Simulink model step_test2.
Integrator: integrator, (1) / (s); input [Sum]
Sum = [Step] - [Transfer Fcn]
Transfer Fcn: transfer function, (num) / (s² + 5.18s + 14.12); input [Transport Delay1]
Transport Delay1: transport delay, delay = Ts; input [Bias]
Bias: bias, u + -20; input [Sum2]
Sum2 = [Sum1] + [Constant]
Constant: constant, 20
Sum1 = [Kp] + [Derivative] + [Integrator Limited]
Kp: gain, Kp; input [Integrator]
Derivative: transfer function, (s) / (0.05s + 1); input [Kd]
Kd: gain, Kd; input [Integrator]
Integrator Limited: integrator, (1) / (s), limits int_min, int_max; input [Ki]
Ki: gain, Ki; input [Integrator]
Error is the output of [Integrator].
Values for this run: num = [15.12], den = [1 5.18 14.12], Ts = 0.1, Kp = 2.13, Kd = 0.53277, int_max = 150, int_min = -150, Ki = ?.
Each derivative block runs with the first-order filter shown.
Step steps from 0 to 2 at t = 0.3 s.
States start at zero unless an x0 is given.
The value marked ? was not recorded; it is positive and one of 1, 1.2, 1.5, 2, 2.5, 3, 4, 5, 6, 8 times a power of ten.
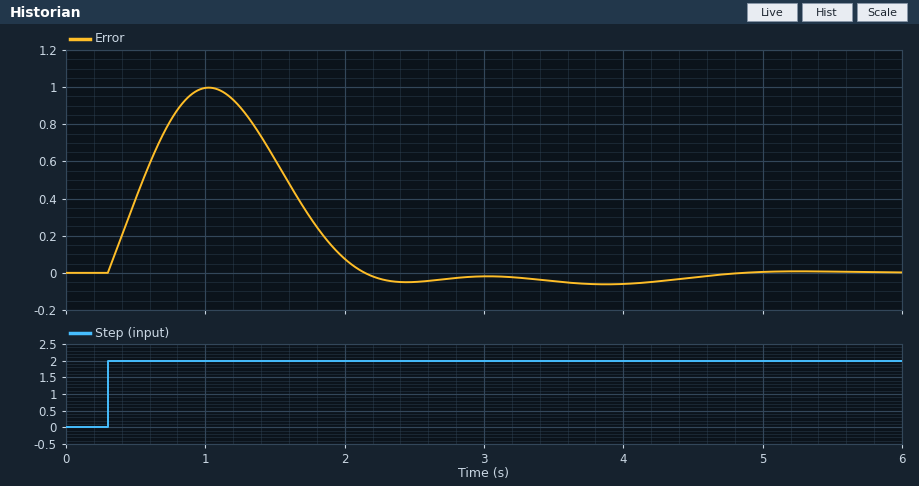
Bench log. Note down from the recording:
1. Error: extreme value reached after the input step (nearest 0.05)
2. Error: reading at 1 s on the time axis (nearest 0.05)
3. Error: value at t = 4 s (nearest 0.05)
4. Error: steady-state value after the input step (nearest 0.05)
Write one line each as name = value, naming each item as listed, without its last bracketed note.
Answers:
Error: extreme value reached after the input step = 1.00
Error: reading at 1 s on the time axis = 1.00
Error: value at t = 4 s = -0.05
Error: steady-state value after the input step = 0.00
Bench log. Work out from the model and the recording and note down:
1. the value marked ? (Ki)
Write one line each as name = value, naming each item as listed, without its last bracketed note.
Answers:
the value marked ? = 2
